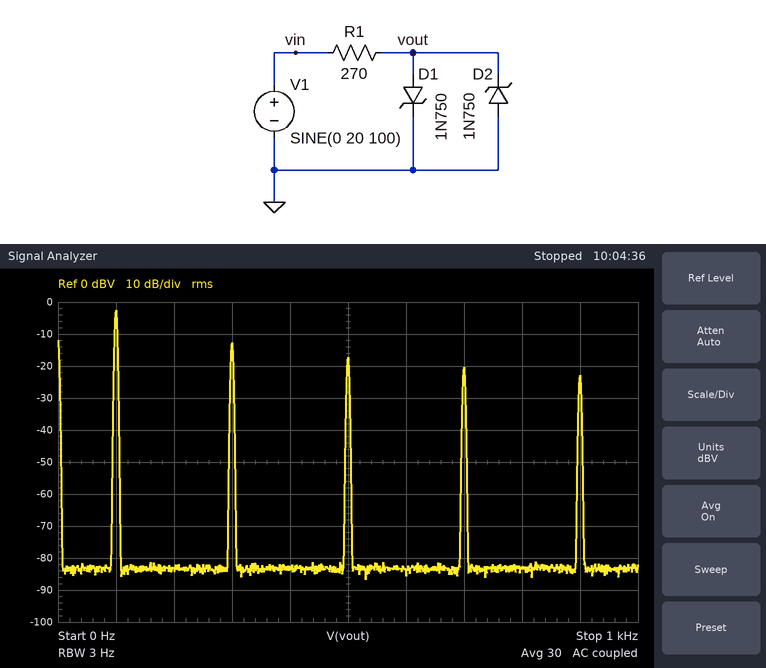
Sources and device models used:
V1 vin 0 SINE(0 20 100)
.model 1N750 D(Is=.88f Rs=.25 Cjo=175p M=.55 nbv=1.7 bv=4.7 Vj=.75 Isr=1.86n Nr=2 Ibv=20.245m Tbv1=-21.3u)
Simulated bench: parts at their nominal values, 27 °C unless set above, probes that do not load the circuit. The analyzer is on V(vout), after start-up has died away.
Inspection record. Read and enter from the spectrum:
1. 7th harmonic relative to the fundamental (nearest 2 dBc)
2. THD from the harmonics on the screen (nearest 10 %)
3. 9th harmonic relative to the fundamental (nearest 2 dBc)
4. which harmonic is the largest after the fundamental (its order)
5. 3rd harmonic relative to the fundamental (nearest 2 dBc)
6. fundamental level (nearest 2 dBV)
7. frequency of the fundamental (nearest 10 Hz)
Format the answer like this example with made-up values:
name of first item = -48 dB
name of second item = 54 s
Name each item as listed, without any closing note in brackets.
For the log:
7th harmonic relative to the fundamental = -18 dBc
THD from the harmonics on the screen = 40 %
9th harmonic relative to the fundamental = -20 dBc
which harmonic is the largest after the fundamental = 3
3rd harmonic relative to the fundamental = -10 dBc
fundamental level = -2 dBV
frequency of the fundamental = 100 Hz
